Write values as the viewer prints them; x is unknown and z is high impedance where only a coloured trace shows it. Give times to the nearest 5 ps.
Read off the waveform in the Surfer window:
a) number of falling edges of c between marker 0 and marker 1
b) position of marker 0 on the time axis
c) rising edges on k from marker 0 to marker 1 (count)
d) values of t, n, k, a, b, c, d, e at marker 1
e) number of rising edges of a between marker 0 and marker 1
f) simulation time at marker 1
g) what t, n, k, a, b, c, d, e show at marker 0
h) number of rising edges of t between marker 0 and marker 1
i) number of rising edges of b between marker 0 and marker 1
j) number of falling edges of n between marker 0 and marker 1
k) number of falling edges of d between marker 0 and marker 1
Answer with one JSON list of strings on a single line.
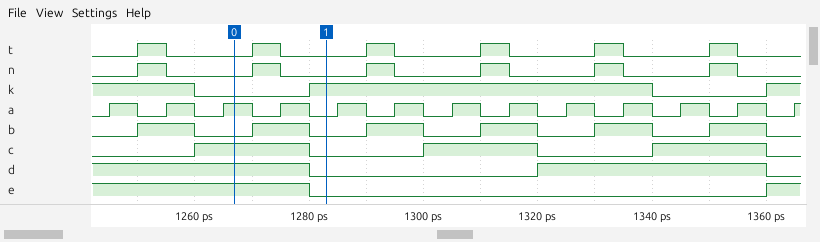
["1", "1265 ps", "1", "t=0, n=0, k=1, a=0, b=0, c=0, d=0, e=0", "1", "1285 ps", "t=0, n=0, k=0, a=1, b=0, c=1, d=1, e=1", "1", "1", "1", "1"]
